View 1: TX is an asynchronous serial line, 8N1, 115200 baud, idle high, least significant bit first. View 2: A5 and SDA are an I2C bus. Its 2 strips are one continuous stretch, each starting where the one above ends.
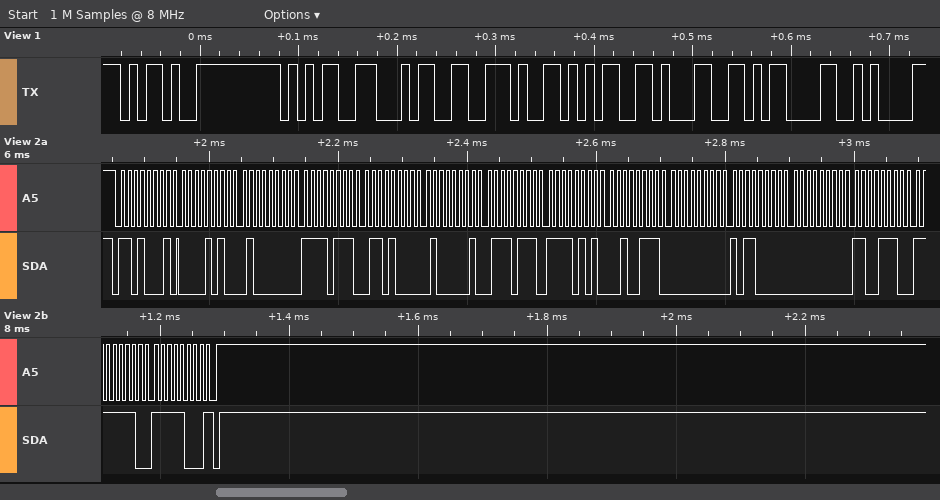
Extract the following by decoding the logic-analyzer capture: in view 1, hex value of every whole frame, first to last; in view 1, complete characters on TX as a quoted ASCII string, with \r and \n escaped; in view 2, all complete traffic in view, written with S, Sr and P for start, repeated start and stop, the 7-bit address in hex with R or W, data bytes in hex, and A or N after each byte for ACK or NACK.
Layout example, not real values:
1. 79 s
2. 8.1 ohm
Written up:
1. 2D 35 34 2E 35 31 0D 0A
2. "-54.51\r\n"
3. S 68R A 0A A 40 A F7 A 68 A 41 A 77 A F5 A 27 A 00 A B0 A 00 A CE A FE A F8 N P
